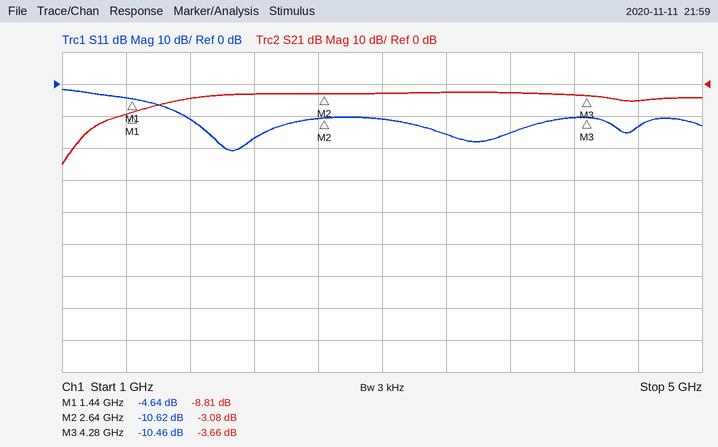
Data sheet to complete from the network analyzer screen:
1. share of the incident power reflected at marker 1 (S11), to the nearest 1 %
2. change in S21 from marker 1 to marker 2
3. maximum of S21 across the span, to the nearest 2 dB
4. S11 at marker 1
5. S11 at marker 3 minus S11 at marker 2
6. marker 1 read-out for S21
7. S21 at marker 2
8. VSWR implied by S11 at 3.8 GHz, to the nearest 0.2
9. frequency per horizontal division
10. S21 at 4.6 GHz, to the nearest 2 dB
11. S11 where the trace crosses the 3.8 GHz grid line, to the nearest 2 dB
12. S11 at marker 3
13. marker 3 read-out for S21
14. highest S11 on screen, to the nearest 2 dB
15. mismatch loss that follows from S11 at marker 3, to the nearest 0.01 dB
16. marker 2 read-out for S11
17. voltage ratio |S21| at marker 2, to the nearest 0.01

34 %
5.73 dB
-2 dB
-4.64 dB
0.16 dB
-8.81 dB
-3.08 dB
1.4
400 MHz
-6 dB
-16 dB
-10.46 dB
-3.66 dB
-2 dB
0.41 dB
-10.62 dB
0.70
